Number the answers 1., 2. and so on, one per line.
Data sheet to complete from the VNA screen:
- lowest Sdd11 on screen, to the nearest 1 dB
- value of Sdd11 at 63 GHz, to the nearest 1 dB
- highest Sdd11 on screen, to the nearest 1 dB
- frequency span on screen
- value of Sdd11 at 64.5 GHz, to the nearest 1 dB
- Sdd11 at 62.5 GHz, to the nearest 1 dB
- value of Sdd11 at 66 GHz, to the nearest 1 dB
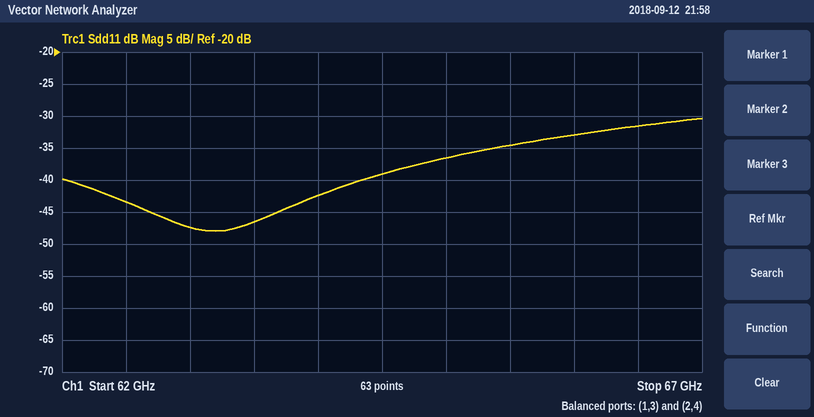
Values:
1. -48 dB
2. -47 dB
3. -30 dB
4. 5 GHz
5. -39 dB
6. -43 dB
7. -33 dB
